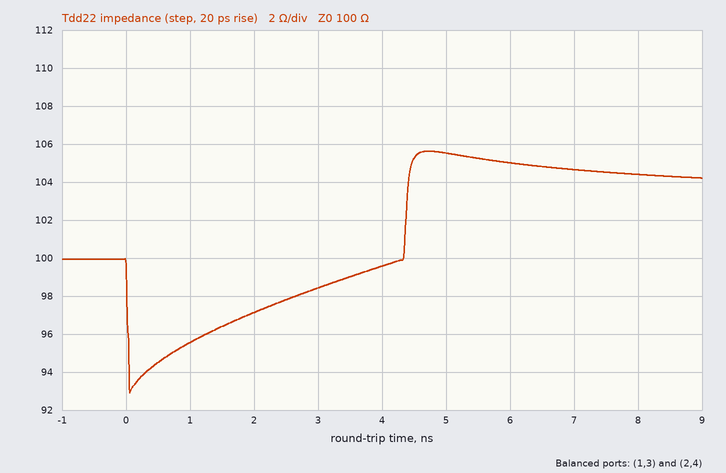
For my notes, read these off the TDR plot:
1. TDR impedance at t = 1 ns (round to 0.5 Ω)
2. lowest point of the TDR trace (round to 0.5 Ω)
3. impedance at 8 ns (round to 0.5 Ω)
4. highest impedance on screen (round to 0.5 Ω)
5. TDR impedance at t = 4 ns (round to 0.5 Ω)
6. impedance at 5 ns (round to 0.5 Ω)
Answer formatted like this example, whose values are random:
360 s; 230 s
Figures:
95.5 Ω; 93.0 Ω; 104.5 Ω; 105.5 Ω; 99.5 Ω; 105.5 Ω
